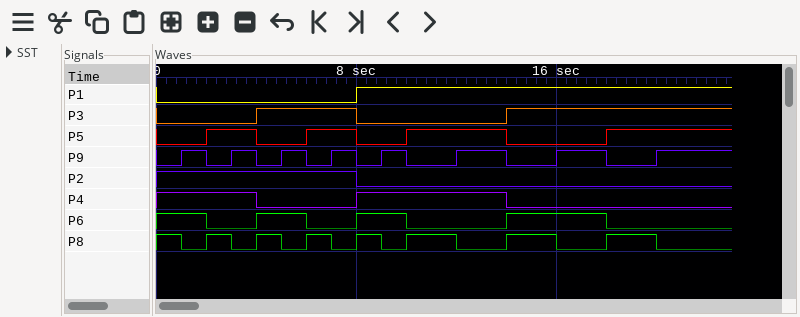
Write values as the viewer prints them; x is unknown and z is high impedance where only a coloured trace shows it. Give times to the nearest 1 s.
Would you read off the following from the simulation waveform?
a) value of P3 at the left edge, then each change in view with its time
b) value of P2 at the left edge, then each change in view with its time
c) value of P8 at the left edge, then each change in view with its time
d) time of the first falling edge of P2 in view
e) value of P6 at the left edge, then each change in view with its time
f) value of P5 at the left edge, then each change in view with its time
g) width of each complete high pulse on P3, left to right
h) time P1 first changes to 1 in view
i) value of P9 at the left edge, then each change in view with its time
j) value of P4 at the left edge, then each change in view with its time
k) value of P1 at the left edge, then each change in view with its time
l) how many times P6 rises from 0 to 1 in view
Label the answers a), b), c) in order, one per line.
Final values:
a) 0, 1 at 4 s, 0 at 8 s, 1 at 14 s
b) 1, 0 at 8 s
c) 1, 0 at 1 s, 1 at 2 s, 0 at 3 s, 1 at 4 s, 0 at 5 s, 1 at 6 s, 0 at 7 s, 1 at 8 s, 0 at 9 s, 1 at 10 s, 0 at 12 s, 1 at 14 s, 0 at 16 s, 1 at 18 s, 0 at 20 s
d) 8 s
e) 1, 0 at 2 s, 1 at 4 s, 0 at 6 s, 1 at 8 s, 0 at 10 s, 1 at 14 s, 0 at 18 s
f) 0, 1 at 2 s, 0 at 4 s, 1 at 6 s, 0 at 8 s, 1 at 10 s, 0 at 14 s, 1 at 18 s
g) 4 s
h) 8 s
i) 0, 1 at 1 s, 0 at 2 s, 1 at 3 s, 0 at 4 s, 1 at 5 s, 0 at 6 s, 1 at 7 s, 0 at 8 s, 1 at 9 s, 0 at 10 s, 1 at 12 s, 0 at 14 s, 1 at 16 s, 0 at 18 s, 1 at 20 s
j) 1, 0 at 4 s, 1 at 8 s, 0 at 14 s
k) 0, 1 at 8 s
l) 3
